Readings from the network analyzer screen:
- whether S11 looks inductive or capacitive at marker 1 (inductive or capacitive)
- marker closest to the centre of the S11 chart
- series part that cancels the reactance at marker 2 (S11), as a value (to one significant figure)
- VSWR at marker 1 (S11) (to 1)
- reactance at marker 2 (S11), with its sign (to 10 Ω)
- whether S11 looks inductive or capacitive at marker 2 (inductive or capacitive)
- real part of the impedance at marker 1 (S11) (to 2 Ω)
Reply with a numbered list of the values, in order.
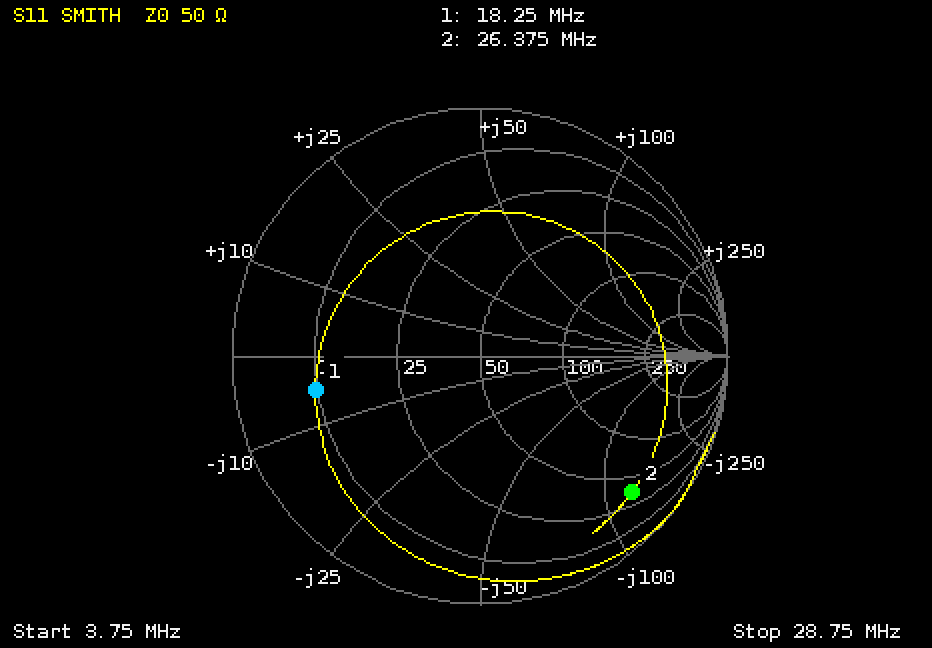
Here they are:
1. capacitive
2. marker 1
3. 700 nH
4. 5
5. -120 Ω
6. capacitive
7. 10 Ω
